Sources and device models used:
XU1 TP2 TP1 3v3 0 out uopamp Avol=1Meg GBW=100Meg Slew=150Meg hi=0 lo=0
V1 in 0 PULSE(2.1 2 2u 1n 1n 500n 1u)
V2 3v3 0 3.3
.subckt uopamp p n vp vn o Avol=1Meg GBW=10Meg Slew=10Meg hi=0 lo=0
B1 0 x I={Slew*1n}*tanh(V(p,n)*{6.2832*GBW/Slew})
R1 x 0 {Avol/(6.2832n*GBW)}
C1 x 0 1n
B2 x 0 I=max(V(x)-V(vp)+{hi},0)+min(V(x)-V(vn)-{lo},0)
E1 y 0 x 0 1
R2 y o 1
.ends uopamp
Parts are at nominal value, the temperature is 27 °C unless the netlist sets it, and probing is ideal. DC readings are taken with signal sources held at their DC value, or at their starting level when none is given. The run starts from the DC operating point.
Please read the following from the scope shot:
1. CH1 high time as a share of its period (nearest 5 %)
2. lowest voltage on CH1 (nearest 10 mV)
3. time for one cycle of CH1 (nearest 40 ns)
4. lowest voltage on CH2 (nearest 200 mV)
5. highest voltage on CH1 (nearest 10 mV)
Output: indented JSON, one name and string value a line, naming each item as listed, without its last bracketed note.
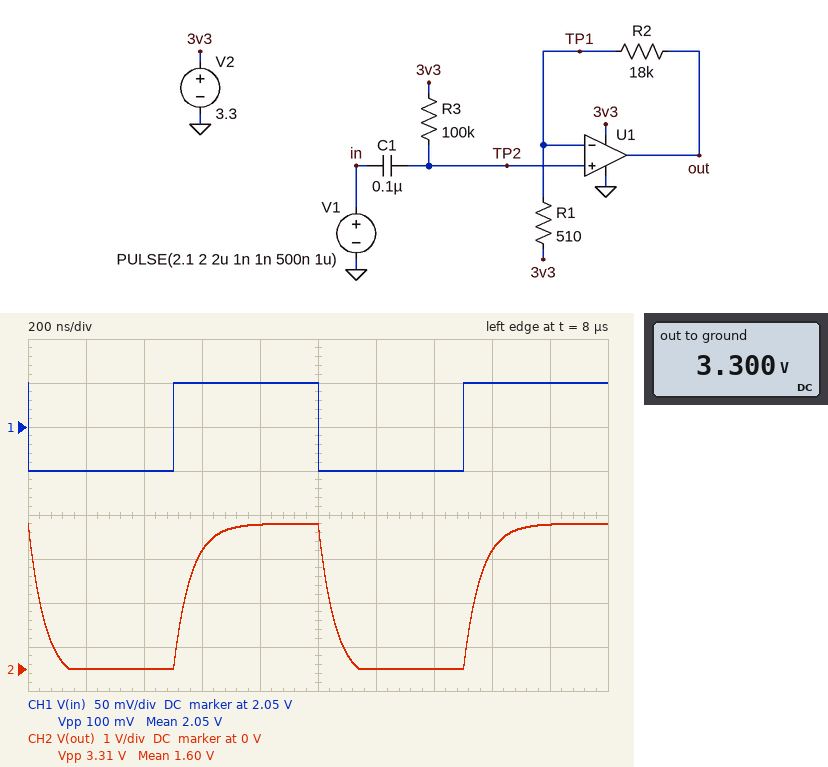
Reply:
{
  "CH1 high time as a share of its period": "50 %",
  "lowest voltage on CH1": "2.00 V",
  "time for one cycle of CH1": "1.00 µs",
  "lowest voltage on CH2": "0 V",
  "highest voltage on CH1": "2.10 V"
}
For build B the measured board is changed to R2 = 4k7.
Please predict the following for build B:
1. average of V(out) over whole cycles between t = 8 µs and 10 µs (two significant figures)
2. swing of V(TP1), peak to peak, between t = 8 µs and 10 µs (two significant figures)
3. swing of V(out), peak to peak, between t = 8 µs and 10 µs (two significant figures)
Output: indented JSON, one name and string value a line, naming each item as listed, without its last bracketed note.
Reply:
{
  "average of V(out) over whole cycles between t = 8 µs and 10 µs": "2.8 V",
  "swing of V(TP1), peak to peak, between t = 8 µs and 10 µs": "100 mV",
  "swing of V(out), peak to peak, between t = 8 µs and 10 µs": "1.0 V"
}
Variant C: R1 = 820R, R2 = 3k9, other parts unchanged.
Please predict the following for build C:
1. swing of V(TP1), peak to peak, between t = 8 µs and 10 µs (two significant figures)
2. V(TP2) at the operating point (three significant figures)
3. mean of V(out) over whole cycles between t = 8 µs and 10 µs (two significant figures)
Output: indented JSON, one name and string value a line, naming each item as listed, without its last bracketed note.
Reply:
{
  "swing of V(TP1), peak to peak, between t = 8 µs and 10 µs": "100 mV",
  "V(TP2) at the operating point": "3.30 V",
  "mean of V(out) over whole cycles between t = 8 µs and 10 µs": "3.0 V"
}
